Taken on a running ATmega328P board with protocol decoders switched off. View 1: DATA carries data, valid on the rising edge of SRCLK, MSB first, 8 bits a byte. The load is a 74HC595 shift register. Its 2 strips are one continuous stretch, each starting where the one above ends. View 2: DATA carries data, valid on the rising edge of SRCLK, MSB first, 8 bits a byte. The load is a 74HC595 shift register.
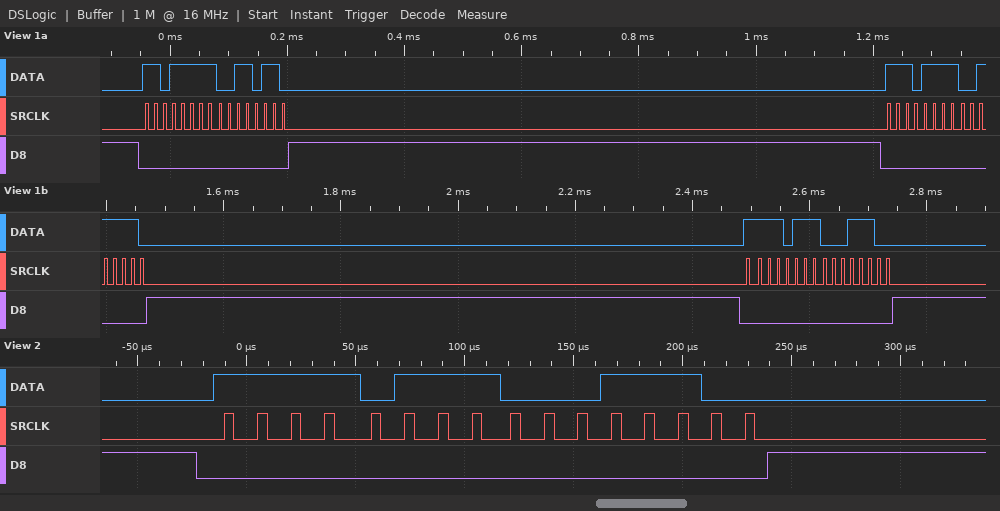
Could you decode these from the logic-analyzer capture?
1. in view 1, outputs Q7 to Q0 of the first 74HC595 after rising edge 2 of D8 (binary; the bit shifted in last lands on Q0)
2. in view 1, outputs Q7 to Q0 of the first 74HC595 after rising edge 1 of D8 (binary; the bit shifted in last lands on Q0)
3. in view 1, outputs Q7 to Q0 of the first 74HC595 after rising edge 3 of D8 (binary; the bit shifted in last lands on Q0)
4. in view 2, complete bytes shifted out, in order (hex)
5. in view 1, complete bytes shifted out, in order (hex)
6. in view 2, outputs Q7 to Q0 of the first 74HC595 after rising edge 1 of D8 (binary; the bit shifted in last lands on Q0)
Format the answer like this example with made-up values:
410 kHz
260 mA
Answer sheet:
00111110
00110110
00011100
F7 1C
DF 36 EF 3E F7 1C
00011100
